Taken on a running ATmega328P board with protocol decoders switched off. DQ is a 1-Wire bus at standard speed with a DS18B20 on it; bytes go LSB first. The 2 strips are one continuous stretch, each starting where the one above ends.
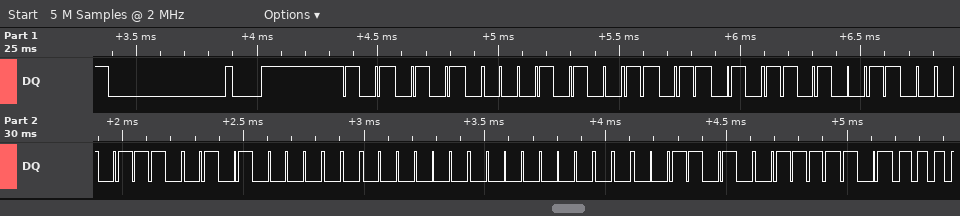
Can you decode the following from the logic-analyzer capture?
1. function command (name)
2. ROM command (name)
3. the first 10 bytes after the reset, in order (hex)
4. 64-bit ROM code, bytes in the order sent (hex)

Read Scratchpad
Match ROM
55 28 5B CB 70 0A 00 00 58 BE
28 5B CB 70 0A 00 00 58
